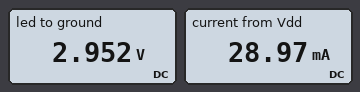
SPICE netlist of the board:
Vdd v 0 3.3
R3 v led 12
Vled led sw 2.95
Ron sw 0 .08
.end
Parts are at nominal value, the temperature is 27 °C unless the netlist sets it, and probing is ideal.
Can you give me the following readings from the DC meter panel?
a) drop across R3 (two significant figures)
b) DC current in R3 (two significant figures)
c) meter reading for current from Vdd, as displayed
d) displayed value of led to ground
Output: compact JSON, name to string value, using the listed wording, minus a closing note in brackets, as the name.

{"drop across R3": "350 mV", "DC current in R3": "29 mA", "meter reading for current from Vdd, as displayed": "28.97 mA", "displayed value of led to ground": "2.952 V"}
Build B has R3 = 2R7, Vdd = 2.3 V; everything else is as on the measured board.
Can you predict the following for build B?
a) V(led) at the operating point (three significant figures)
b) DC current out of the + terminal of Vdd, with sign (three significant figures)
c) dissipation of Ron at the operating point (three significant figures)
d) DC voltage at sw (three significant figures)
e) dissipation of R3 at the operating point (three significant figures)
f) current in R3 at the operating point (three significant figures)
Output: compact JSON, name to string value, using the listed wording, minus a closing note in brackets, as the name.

{"V(led) at the operating point": "2.93 V", "DC current out of the + terminal of Vdd, with sign": "-234 mA", "dissipation of Ron at the operating point": "4.37 mW", "DC voltage at sw": "-18.7 mV", "dissipation of R3 at the operating point": "148 mW", "current in R3 at the operating point": "234 mA"}
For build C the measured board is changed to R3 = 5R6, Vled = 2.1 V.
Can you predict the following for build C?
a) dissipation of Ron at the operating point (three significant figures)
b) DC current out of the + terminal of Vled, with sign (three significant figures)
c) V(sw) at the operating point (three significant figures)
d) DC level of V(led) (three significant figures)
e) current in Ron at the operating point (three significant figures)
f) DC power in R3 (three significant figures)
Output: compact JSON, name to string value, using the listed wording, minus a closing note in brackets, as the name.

{"dissipation of Ron at the operating point": "3.57 mW", "DC current out of the + terminal of Vled, with sign": "-211 mA", "V(sw) at the operating point": "16.9 mV", "DC level of V(led)": "2.12 V", "current in Ron at the operating point": "211 mA", "DC power in R3": "250 mW"}
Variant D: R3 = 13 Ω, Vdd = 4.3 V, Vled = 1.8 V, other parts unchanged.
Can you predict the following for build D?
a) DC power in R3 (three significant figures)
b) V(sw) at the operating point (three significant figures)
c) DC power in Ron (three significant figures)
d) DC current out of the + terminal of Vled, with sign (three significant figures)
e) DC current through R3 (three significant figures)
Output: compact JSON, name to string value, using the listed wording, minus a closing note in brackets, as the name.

{"DC power in R3": "475 mW", "V(sw) at the operating point": "15.3 mV", "DC power in Ron": "2.92 mW", "DC current out of the + terminal of Vled, with sign": "-191 mA", "DC current through R3": "191 mA"}
